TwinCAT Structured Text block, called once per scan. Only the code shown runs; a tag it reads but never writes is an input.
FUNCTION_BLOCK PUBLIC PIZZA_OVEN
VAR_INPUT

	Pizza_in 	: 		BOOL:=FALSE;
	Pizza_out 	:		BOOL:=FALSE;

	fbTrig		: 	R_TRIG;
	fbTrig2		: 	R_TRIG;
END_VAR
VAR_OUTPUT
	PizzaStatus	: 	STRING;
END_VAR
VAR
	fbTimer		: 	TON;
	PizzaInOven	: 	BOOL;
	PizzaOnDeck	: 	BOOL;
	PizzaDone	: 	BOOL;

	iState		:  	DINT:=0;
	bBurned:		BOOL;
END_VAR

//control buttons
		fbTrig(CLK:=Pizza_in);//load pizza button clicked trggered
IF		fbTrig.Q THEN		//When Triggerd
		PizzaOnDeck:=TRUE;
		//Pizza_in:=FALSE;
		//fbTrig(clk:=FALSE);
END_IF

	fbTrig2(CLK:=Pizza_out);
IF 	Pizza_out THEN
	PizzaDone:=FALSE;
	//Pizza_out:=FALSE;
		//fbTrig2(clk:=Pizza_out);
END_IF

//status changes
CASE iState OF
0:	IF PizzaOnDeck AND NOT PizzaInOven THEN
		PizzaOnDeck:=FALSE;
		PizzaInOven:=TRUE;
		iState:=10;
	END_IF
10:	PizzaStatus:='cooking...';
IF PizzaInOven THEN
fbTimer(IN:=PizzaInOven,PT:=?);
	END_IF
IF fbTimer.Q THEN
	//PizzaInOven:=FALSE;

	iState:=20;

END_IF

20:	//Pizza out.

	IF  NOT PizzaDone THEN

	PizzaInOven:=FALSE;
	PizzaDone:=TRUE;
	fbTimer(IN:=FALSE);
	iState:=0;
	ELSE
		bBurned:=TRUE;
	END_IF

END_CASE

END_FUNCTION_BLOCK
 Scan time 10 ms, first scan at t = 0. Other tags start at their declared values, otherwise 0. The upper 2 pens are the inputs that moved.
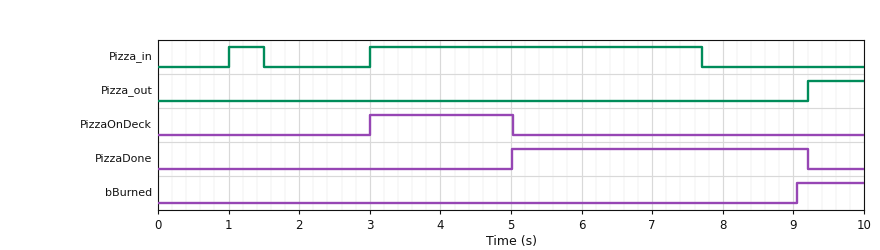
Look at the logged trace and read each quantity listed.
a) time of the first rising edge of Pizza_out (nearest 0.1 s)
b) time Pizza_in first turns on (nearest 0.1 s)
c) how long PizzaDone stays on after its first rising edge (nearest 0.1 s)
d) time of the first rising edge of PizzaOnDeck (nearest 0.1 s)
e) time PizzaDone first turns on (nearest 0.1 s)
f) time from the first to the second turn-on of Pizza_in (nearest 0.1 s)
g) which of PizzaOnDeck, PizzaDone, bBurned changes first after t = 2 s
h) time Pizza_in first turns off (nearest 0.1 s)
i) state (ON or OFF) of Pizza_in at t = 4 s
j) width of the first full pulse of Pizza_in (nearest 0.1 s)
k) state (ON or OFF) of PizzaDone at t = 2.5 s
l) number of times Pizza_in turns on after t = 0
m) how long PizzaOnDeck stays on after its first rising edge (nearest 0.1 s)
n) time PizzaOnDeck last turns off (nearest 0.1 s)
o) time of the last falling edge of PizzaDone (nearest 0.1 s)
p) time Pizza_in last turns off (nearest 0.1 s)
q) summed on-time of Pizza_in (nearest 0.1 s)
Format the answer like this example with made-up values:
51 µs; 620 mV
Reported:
9.2 s; 1.0 s; 4.2 s; 3.0 s; 5.0 s; 2.0 s; PizzaOnDeck; 1.5 s; ON; 0.5 s; OFF; 2; 2.0 s; 5.0 s; 9.2 s; 7.7 s; 5.2 s
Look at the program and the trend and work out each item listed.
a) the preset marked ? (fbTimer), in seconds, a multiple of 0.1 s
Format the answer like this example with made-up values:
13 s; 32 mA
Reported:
4.0 s
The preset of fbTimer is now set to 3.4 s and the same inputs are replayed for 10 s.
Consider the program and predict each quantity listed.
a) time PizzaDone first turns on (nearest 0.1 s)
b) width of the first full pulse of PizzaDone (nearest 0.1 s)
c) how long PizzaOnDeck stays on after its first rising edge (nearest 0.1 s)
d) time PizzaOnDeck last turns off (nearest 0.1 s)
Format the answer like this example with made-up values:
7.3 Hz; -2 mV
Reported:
4.4 s; 4.8 s; 1.4 s; 4.4 s
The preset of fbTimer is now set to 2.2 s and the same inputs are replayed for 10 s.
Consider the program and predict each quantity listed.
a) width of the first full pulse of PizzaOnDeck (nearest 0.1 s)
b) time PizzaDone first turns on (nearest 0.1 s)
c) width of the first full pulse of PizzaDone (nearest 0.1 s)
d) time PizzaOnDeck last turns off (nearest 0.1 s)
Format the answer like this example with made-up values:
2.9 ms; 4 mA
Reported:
0.2 s; 3.2 s; 6.0 s; 3.2 s
